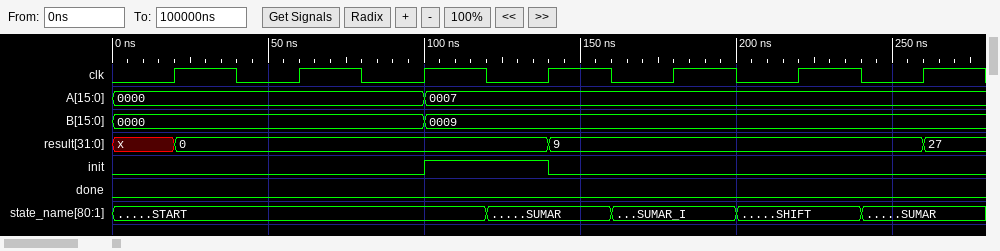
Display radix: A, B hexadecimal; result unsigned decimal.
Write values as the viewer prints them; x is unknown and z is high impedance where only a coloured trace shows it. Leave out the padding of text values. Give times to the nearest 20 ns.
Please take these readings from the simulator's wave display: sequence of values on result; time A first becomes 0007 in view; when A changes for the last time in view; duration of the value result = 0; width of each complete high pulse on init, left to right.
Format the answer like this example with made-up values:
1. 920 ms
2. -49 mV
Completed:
1. x, 0, 9, 27
2. 100 ns
3. 100 ns
4. 120 ns
5. 40 ns
